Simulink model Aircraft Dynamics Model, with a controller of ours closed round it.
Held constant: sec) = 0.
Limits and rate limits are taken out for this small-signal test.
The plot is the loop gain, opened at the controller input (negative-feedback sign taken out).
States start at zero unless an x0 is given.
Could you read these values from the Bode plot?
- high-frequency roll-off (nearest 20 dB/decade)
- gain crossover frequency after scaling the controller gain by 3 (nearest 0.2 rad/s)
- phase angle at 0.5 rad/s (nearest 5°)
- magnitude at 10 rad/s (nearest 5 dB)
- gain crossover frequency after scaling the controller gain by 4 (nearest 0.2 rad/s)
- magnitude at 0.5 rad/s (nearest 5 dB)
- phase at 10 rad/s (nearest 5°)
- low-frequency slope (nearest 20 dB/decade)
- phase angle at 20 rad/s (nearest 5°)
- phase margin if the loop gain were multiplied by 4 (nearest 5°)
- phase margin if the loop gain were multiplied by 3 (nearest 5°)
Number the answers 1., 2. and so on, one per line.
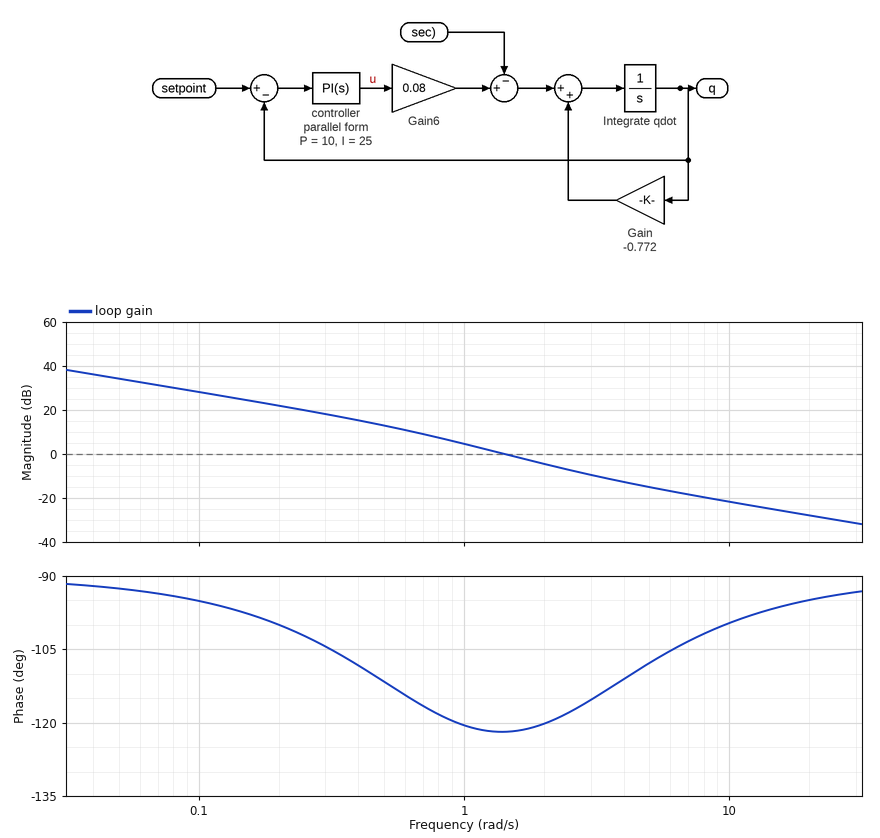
1. -20 dB/decade
2. 3.0 rad/s
3. -110°
4. -20 dB
5. 3.8 rad/s
6. 15 dB
7. -100°
8. -20 dB/decade
9. -95°
10. 70°
11. 65°
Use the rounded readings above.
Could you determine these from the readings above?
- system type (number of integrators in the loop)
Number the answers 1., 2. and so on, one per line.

1. 1
